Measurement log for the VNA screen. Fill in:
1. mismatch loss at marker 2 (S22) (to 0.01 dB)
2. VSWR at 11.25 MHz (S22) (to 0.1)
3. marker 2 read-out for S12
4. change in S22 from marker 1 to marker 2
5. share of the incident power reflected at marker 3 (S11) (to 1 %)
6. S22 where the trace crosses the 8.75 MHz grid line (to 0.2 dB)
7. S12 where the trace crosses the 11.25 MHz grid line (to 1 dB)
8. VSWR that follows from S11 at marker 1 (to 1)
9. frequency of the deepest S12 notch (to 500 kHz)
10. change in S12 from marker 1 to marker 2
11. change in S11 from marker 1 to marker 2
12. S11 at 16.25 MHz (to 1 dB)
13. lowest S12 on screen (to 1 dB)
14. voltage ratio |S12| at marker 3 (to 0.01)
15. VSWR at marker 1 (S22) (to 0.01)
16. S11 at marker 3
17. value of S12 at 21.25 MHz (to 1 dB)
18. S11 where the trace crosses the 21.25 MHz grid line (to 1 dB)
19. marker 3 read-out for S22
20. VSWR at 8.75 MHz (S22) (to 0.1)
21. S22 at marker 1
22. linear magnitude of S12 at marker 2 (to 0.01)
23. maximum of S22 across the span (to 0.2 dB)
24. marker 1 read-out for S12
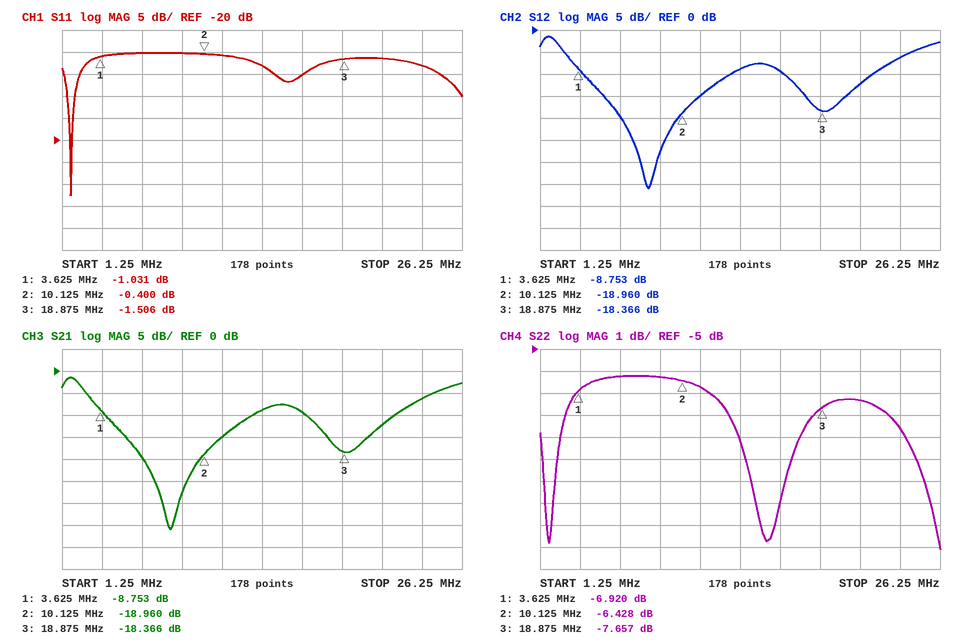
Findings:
1.12 dB
2.7
-18.960 dB
0.492 dB
71 %
-6.2 dB
-15 dB
17
8.0 MHz
-10.207 dB
0.631 dB
-5 dB
-36 dB
0.12
2.64
-1.506 dB
-12 dB
-1 dB
-7.657 dB
2.9
-6.920 dB
0.11
-6.2 dB
-8.753 dB
